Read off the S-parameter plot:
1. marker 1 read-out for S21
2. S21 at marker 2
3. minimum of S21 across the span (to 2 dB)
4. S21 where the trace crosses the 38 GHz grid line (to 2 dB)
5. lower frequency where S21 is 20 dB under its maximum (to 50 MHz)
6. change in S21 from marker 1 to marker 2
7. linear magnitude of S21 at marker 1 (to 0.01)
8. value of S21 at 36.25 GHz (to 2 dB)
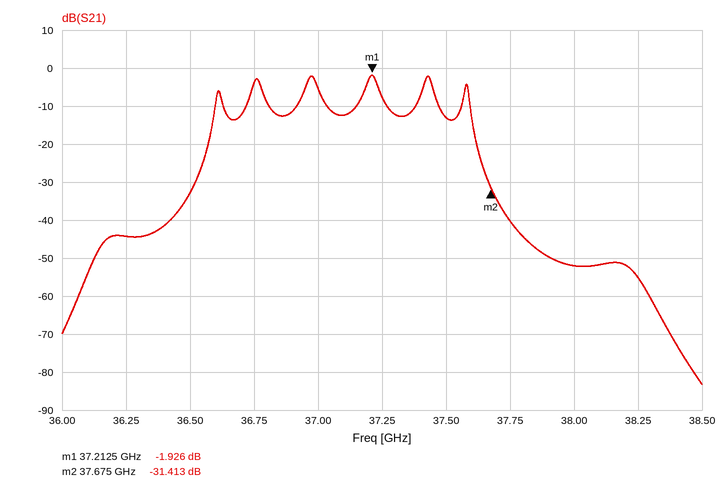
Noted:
-1.926 dB
-31.413 dB
-84 dB
-52 dB
36.55 GHz
-29.487 dB
0.80
-44 dB
